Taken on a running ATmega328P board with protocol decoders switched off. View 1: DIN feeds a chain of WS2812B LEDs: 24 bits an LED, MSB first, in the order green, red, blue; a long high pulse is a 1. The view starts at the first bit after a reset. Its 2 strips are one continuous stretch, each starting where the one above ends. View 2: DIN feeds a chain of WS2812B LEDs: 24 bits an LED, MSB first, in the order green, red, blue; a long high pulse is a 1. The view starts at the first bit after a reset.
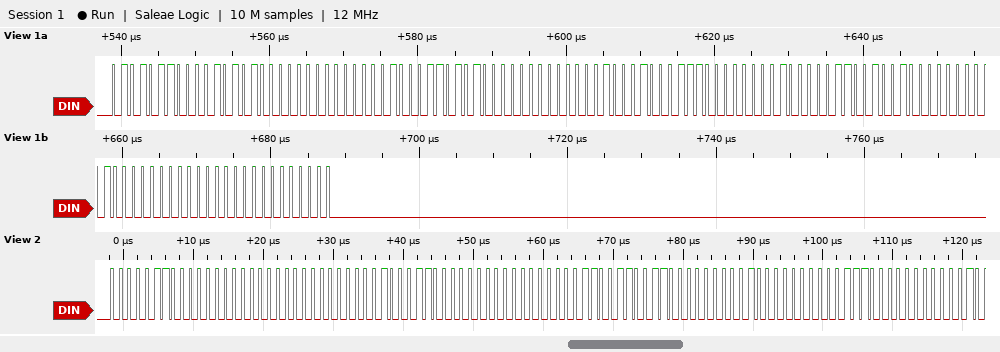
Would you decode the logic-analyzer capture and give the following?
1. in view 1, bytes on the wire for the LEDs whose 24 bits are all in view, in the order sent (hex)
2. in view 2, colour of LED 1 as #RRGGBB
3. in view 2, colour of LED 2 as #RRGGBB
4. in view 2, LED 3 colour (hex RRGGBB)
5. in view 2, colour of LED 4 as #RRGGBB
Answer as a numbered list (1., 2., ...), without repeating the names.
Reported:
1. 56 15 00 02 35 00 04 47 00 83 24 01 00 00 00
2. #000600
3. #180100
4. #330300
5. #0E4000
